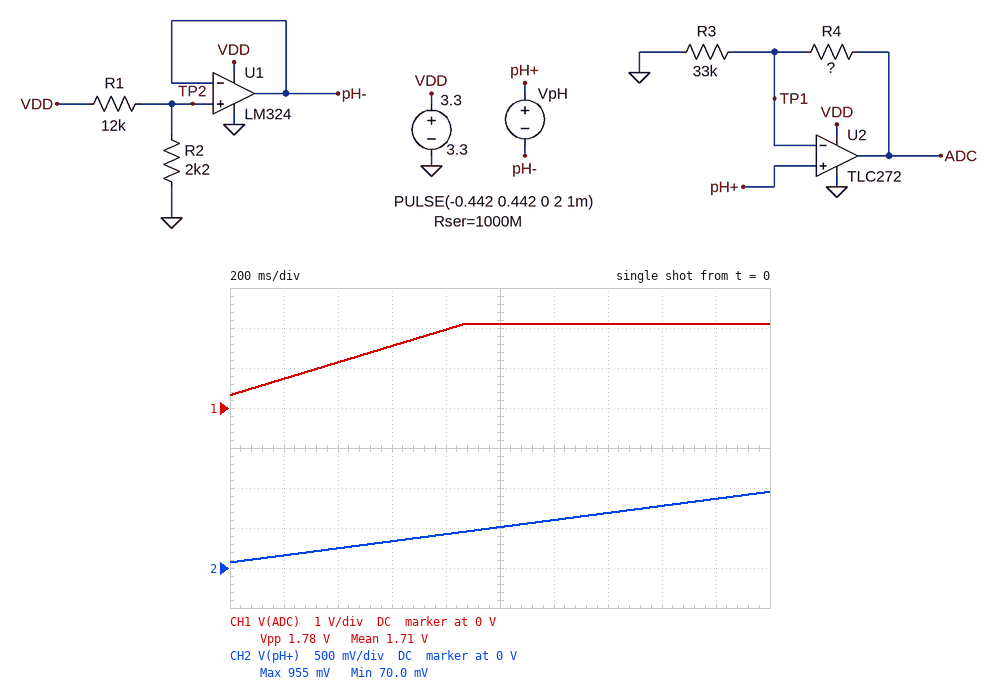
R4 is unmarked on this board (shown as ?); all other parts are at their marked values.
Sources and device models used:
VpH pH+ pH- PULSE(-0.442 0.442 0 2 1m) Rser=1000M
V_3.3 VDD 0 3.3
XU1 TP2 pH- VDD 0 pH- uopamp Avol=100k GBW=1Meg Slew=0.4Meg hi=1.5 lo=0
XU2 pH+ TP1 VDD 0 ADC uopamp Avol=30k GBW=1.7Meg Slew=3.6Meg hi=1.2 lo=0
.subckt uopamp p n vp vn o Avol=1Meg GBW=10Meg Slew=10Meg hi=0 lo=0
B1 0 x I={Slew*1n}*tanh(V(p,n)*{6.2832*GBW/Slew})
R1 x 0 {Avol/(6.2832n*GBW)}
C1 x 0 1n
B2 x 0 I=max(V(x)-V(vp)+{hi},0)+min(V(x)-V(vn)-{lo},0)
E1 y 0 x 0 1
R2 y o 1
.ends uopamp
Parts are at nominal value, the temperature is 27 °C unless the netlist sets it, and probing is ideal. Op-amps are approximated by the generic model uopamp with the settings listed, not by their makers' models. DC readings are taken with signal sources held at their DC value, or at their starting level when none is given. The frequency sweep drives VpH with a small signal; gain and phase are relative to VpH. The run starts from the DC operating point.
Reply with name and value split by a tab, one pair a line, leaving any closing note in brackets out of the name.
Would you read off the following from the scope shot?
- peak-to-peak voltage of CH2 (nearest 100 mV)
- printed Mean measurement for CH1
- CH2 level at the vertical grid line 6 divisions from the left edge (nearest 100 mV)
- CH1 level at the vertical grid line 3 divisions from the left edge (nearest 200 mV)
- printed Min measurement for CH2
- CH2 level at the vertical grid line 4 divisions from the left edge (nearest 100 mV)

peak-to-peak voltage of CH2	900 mV
printed Mean measurement for CH1	1.71 V
CH2 level at the vertical grid line 6 divisions from the left edge	600 mV
CH1 level at the vertical grid line 3 divisions from the left edge	1.6 V
printed Min measurement for CH2	70.0 mV
CH2 level at the vertical grid line 4 divisions from the left edge	400 mV
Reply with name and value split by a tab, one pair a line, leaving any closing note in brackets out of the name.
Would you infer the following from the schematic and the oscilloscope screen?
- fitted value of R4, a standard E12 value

fitted value of R4, a standard E12 value	120 kΩ
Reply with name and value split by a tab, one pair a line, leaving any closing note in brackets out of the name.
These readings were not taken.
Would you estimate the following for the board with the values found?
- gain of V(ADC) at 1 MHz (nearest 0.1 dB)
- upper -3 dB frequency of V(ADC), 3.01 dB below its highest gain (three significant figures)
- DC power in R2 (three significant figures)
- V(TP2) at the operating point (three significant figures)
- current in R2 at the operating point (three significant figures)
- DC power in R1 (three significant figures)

gain of V(ADC) at 1 MHz	4.1 dB
upper -3 dB frequency of V(ADC), 3.01 dB below its highest gain	367 kHz
DC power in R2	119 µW
V(TP2) at the operating point	511 mV
current in R2 at the operating point	232 µA
DC power in R1	648 µW
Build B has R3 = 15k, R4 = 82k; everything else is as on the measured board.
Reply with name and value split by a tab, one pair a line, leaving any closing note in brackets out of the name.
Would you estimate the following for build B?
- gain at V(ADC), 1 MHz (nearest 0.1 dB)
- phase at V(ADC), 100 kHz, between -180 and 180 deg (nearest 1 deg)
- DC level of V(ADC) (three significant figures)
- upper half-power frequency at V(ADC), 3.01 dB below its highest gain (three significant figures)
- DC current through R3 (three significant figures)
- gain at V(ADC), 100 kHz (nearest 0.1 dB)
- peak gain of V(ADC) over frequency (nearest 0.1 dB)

gain at V(ADC), 1 MHz	4.3 dB
phase at V(ADC), 100 kHz, between -180 and 180 deg	-21 deg
DC level of V(ADC)	448 mV
upper half-power frequency at V(ADC), 3.01 dB below its highest gain	263 kHz
DC current through R3	4.62 µA
gain at V(ADC), 100 kHz	15.6 dB
peak gain of V(ADC) over frequency	16.2 dB
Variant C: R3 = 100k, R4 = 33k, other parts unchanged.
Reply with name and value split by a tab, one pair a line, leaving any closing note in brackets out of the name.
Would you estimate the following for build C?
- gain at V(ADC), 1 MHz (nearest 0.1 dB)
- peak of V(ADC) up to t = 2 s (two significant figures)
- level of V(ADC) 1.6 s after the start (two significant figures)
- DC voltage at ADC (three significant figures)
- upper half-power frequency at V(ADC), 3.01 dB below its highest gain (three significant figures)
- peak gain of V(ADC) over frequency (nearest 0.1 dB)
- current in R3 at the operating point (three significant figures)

gain at V(ADC), 1 MHz	0.4 dB
peak of V(ADC) up to t = 2 s	1.3 V
level of V(ADC) 1.6 s after the start	1.0 V
DC voltage at ADC	92.1 mV
upper half-power frequency at V(ADC), 3.01 dB below its highest gain	1.28 MHz
peak gain of V(ADC) over frequency	2.5 dB
current in R3 at the operating point	693 nA
